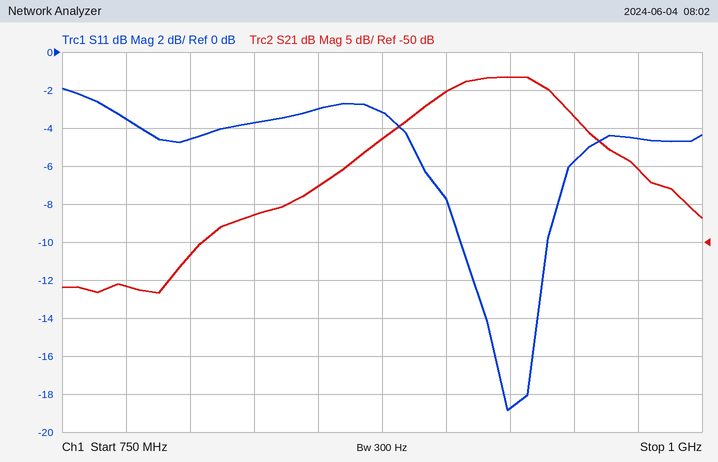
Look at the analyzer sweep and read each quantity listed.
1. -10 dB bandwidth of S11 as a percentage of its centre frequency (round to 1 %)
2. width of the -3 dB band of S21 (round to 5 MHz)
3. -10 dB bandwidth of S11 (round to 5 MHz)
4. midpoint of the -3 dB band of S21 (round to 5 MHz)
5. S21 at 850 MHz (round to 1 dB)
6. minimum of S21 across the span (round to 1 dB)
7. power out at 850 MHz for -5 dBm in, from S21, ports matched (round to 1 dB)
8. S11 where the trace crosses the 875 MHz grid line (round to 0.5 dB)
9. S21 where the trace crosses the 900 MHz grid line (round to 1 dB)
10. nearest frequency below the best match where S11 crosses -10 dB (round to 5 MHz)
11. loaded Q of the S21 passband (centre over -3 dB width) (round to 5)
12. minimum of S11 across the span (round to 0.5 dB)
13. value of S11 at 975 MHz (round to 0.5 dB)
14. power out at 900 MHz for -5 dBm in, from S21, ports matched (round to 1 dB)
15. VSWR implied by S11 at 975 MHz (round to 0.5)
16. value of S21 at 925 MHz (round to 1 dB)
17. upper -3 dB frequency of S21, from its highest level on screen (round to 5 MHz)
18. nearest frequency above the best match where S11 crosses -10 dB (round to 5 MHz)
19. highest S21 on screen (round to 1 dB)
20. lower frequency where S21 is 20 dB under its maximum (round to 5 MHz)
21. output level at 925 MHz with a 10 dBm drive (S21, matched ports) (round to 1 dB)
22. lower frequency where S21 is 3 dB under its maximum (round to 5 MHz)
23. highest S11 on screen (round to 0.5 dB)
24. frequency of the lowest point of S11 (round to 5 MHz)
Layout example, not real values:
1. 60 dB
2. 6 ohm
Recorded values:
1. 4 %
2. 50 MHz
3. 35 MHz
4. 920 MHz
5. -43 dB
6. -57 dB
7. -48 dBm
8. -3.0 dB
9. -30 dB
10. 905 MHz
11. 20
12. -19.0 dB
13. -4.5 dB
14. -35 dBm
15. 4.0
16. -28 dB
17. 945 MHz
18. 940 MHz
19. -28 dB
20. 810 MHz
21. -18 dBm
22. 895 MHz
23. -2.0 dB
24. 925 MHz
